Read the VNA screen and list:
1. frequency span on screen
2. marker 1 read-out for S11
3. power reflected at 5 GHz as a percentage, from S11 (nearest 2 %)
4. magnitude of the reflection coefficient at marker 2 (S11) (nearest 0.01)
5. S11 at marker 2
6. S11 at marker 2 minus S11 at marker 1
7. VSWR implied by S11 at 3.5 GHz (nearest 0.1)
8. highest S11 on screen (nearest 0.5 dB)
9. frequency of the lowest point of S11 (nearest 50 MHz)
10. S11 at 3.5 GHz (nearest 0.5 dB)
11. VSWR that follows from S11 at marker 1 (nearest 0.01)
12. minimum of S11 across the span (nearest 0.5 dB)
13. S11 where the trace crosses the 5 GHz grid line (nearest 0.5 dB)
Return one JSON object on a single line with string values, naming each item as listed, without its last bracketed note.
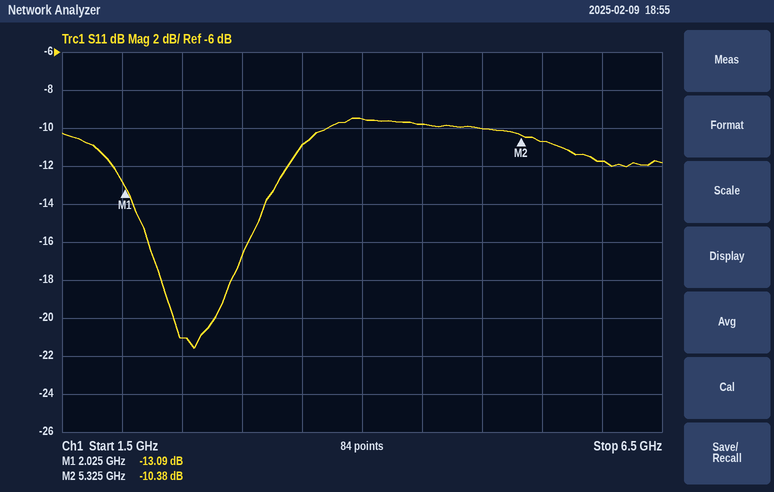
{"frequency span on screen": "5 GHz", "marker 1 read-out for S11": "-13.09 dB", "power reflected at 5 GHz as a percentage, from S11": "10 %", "magnitude of the reflection coefficient at marker 2 (S11)": "0.30", "S11 at marker 2": "-10.38 dB", "S11 at marker 2 minus S11 at marker 1": "2.71 dB", "VSWR implied by S11 at 3.5 GHz": "1.8", "highest S11 on screen": "-9.5 dB", "frequency of the lowest point of S11": "2.60 GHz", "S11 at 3.5 GHz": "-11.0 dB", "VSWR that follows from S11 at marker 1": "1.57", "minimum of S11 across the span": "-21.5 dB", "S11 where the trace crosses the 5 GHz grid line": "-10.0 dB"}
